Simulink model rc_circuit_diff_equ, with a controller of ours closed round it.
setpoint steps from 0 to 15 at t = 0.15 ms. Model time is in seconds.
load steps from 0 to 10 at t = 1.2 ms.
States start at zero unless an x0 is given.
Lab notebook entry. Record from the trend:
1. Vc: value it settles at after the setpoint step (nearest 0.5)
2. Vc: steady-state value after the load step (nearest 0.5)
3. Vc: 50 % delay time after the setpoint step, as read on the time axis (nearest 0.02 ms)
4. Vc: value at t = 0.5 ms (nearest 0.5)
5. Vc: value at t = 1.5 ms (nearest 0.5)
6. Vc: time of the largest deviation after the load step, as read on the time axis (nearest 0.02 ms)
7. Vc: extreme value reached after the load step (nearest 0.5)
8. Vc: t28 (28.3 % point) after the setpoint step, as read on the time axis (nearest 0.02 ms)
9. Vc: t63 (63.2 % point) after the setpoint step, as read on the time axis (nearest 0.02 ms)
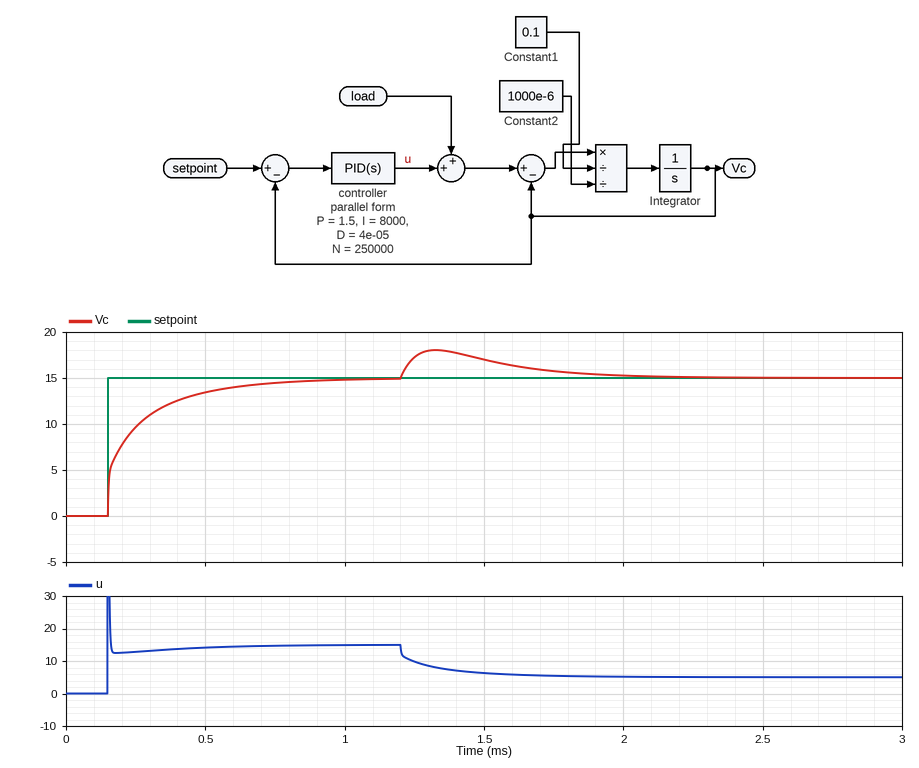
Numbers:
15.0
15.0
0.20 ms
13.5
17.0
1.32 ms
18.0
0.16 ms
0.24 ms
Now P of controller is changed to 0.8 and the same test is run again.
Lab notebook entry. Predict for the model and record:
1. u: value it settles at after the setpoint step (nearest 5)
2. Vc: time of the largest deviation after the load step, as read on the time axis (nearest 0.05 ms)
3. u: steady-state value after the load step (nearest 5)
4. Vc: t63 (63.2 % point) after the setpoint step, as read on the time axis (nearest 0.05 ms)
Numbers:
15
1.35 ms
5
0.30 ms
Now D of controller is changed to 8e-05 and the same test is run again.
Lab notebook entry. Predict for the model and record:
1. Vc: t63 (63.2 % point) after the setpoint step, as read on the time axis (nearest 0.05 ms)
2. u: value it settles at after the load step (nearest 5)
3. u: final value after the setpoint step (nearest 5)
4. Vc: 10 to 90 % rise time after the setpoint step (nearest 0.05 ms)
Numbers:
0.25 ms
5
15
0.40 ms
